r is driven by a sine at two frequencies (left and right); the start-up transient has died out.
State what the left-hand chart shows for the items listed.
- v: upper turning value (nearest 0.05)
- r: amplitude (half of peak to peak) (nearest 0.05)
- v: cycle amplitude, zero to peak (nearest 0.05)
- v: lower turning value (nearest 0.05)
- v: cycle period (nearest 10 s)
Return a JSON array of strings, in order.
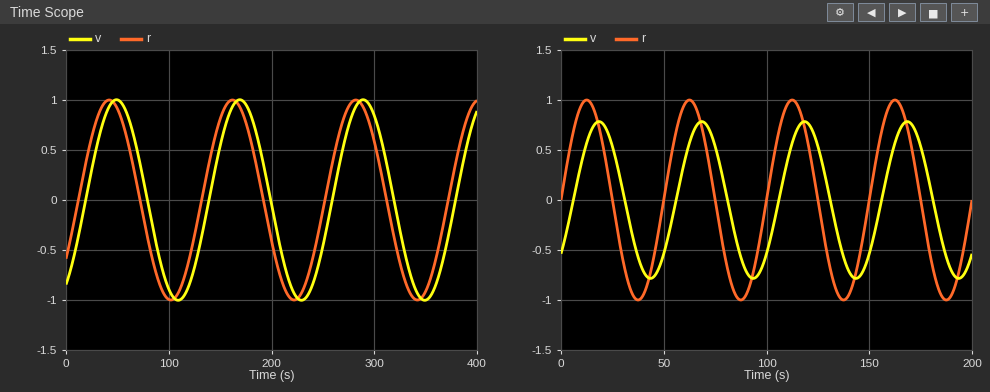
["1.00", "1.00", "1.00", "-1.00", "120 s"]
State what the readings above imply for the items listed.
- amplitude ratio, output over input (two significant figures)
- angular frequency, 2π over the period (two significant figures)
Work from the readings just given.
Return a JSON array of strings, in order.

["1.0", "0.052 rad/s"]
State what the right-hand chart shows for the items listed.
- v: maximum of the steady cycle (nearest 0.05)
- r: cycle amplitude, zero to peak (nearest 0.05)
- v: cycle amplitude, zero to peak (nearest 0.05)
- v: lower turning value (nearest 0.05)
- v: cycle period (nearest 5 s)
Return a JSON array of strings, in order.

["0.80", "1.00", "0.80", "-0.80", "50 s"]
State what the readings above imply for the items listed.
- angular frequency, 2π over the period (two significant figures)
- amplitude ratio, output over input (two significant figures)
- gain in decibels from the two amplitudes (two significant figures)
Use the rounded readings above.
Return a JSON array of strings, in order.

["0.13 rad/s", "0.80", "-1.9 dB"]
